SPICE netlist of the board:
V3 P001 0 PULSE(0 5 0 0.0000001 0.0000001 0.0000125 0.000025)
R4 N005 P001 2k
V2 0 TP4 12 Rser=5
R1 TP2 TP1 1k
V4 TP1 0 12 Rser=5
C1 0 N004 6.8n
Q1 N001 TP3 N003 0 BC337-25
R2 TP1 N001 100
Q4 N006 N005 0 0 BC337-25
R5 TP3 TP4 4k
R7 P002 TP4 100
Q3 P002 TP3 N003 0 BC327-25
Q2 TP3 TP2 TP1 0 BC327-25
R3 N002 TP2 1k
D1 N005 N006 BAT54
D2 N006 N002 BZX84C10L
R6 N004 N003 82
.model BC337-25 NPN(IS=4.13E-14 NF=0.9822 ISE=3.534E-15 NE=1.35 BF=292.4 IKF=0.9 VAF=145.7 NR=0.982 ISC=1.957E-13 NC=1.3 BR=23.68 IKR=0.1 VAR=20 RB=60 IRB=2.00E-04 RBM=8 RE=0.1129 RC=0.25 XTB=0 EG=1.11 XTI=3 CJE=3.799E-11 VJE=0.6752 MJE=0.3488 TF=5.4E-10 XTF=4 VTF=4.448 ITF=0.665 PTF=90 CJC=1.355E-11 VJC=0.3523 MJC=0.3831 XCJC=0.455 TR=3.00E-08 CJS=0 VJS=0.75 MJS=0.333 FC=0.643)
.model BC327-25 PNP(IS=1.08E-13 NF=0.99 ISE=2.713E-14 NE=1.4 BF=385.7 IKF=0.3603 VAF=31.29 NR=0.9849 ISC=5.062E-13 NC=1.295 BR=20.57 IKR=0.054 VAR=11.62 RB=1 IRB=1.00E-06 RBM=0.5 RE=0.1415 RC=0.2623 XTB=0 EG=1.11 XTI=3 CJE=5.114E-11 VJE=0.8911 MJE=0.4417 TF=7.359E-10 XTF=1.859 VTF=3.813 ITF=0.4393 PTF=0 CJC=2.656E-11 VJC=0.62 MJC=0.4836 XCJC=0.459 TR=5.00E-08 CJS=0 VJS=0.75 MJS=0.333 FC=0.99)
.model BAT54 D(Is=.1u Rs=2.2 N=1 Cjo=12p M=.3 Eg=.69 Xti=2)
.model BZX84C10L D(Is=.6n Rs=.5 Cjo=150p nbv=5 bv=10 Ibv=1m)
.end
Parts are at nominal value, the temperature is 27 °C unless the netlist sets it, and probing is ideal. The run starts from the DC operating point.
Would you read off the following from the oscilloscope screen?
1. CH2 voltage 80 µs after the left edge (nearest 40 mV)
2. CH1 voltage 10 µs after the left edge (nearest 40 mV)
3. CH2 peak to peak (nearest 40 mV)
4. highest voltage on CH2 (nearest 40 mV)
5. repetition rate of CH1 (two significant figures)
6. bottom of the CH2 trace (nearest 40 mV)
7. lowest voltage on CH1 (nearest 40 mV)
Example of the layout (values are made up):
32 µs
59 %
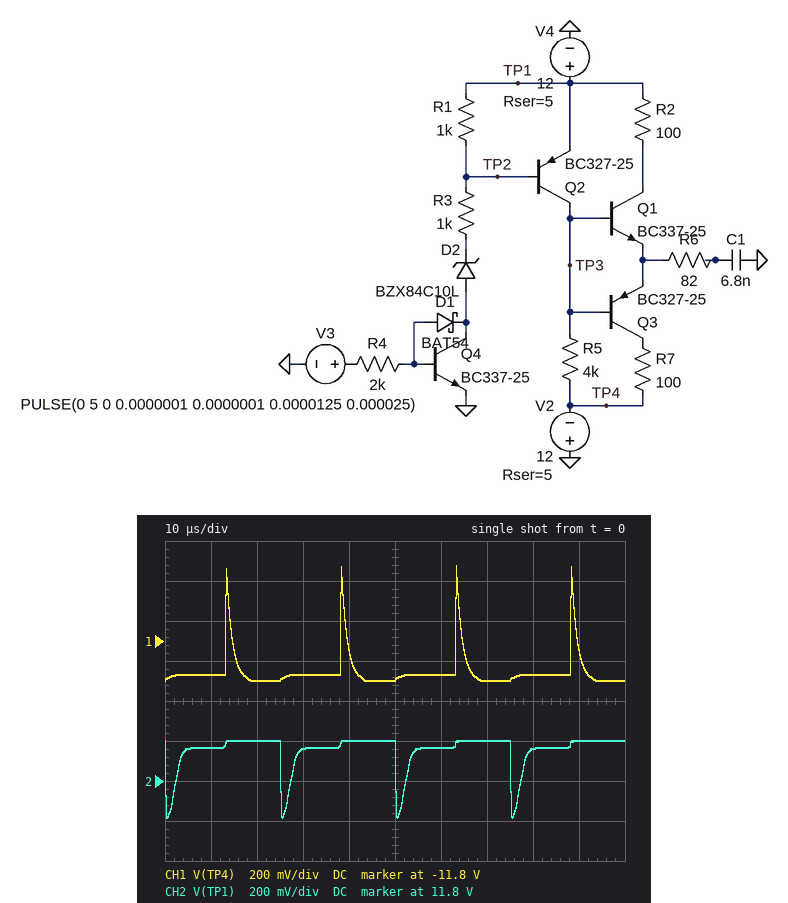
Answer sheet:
11.96 V
-11.96 V
400 mV
12.00 V
40 kHz
11.60 V
-12.00 V
